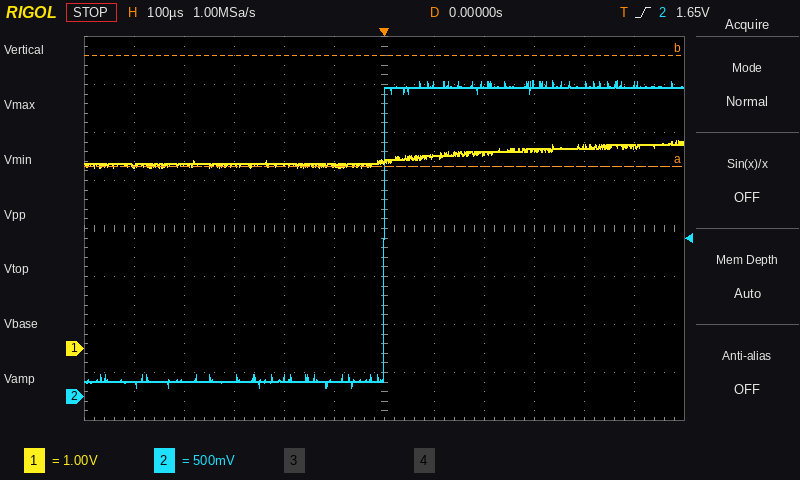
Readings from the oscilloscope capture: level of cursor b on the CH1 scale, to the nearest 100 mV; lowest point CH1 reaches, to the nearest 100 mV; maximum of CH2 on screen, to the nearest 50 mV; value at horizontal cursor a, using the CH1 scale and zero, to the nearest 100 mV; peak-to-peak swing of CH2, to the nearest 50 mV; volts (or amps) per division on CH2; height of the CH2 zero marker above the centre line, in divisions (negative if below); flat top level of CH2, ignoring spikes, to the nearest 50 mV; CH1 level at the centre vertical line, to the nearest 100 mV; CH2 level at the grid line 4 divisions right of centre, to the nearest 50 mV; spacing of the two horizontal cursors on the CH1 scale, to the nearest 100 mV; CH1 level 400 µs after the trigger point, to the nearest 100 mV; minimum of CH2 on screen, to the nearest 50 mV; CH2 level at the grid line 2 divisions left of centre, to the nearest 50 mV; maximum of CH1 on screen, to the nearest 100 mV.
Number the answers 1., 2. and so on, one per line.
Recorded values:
1. 6.1 V
2. 3.8 V
3. 3.30 V
4. 3.8 V
5. 3.20 V
6. 500 mV
7. -3.5 div
8. 3.20 V
9. 3.9 V
10. 3.25 V
11. 2.3 V
12. 4.2 V
13. 100 mV
14. 200 mV
15. 4.3 V
